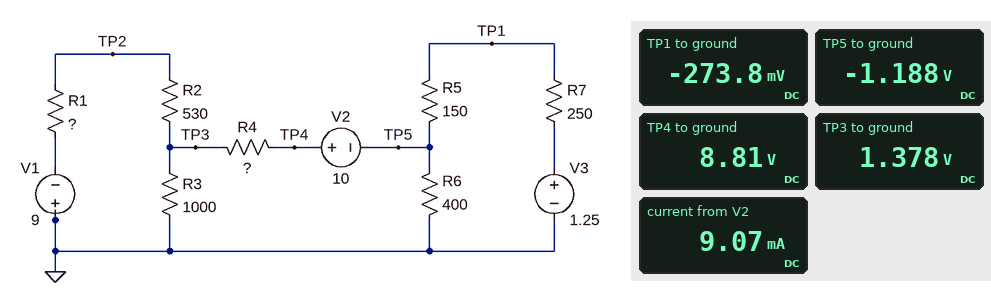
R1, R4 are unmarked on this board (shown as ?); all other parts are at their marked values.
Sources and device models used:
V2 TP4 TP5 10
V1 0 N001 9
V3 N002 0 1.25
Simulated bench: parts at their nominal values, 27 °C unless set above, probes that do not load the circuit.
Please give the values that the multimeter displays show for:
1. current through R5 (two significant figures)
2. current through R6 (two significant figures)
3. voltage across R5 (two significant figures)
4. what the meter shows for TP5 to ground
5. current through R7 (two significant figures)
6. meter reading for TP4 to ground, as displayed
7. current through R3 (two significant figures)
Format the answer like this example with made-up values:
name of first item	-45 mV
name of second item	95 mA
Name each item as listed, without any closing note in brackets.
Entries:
current through R5	6.1 mA
current through R6	3.0 mA
voltage across R5	910 mV
what the meter shows for TP5 to ground	-1.188 V
current through R7	6.1 mA
meter reading for TP4 to ground, as displayed	8.81 V
current through R3	1.4 mA
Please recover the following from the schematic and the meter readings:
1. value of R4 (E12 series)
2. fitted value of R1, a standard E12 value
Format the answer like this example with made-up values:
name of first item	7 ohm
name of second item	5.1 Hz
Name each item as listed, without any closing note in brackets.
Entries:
value of R4	820 Ω
fitted value of R1, a standard E12 value	820 Ω
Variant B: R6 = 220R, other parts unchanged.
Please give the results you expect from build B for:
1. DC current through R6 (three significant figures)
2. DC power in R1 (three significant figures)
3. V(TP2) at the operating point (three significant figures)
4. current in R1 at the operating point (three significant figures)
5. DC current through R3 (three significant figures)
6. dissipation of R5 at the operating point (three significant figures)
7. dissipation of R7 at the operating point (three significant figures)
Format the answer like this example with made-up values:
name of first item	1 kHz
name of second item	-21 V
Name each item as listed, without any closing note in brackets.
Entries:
DC current through R6	3.98 mA
DC power in R1	49.7 mW
V(TP2) at the operating point	-2.62 V
current in R1 at the operating point	7.78 mA
DC current through R3	1.51 mA
dissipation of R5 at the operating point	4.23 mW
dissipation of R7 at the operating point	7.06 mW
